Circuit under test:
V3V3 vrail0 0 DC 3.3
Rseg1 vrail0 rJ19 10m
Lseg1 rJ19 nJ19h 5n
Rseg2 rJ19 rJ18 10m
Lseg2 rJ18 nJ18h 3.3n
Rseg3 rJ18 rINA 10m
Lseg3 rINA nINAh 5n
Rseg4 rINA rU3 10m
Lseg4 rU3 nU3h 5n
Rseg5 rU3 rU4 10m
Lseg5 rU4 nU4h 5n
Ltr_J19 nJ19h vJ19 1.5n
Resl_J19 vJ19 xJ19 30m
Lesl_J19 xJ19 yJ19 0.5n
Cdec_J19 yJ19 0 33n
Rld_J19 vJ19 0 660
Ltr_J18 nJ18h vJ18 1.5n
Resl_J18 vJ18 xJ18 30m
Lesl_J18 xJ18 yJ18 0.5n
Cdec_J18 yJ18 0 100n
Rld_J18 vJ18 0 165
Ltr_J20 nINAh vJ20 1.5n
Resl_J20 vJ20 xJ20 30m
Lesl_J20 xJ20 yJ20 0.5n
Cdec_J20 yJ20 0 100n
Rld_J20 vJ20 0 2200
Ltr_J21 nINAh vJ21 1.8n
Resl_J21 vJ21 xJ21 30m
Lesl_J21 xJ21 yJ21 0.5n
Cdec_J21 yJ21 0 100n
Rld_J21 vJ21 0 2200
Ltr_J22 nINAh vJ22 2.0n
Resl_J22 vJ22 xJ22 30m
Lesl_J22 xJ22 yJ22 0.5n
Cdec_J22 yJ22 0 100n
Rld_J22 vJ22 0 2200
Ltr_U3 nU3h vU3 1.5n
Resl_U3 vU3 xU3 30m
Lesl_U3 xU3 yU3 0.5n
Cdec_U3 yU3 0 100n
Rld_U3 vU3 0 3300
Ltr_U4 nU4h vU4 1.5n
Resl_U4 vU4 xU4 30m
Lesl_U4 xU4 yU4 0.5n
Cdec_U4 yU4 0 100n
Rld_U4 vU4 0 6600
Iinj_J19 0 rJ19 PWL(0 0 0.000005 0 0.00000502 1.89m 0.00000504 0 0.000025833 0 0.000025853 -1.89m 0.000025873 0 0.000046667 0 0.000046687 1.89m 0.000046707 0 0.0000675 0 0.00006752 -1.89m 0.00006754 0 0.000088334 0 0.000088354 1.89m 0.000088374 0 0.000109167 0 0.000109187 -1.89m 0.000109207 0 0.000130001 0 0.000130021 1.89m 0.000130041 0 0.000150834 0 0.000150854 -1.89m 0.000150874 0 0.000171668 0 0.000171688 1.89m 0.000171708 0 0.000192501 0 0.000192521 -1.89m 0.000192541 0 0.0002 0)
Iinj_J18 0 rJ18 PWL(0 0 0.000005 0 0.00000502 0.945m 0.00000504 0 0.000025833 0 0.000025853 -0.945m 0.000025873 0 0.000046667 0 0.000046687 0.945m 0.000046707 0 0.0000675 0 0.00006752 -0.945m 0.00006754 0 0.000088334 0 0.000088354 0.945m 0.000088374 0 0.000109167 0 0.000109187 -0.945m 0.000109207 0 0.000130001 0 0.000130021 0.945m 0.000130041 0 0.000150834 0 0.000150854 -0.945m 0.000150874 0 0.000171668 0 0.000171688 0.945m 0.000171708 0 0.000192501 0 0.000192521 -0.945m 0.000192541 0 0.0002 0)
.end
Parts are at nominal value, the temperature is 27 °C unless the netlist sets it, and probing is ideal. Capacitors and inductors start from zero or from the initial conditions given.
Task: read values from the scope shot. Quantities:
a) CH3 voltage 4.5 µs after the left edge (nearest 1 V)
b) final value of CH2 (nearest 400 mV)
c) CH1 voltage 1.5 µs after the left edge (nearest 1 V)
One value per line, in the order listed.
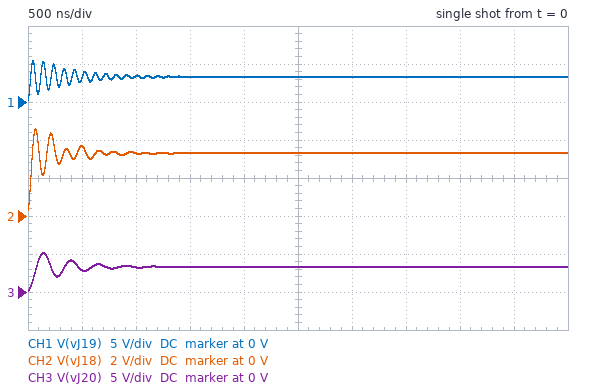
3 V
3.2 V
3 V
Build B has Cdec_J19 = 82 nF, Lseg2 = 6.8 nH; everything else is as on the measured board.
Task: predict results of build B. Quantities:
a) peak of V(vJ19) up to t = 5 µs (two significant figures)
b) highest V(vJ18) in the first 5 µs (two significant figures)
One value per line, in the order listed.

5.2 V
4.8 V
